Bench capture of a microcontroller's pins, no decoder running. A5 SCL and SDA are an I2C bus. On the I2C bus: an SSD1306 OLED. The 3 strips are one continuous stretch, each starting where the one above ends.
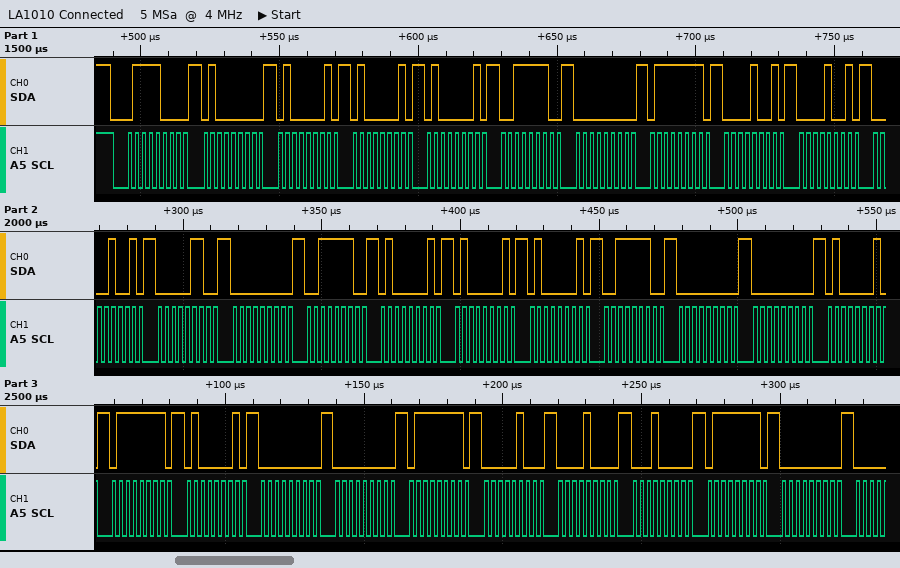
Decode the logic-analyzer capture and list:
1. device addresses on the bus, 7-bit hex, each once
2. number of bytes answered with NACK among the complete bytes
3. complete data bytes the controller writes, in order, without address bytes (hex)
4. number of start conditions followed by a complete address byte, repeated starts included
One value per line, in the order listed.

0x3C
0
40 41 41 41 3E 00 7F 09 09 09 06 00 3E 41 41 41 3E 00 00 41 7F 41 00 00 7F 04 08 10 7F 00
1
